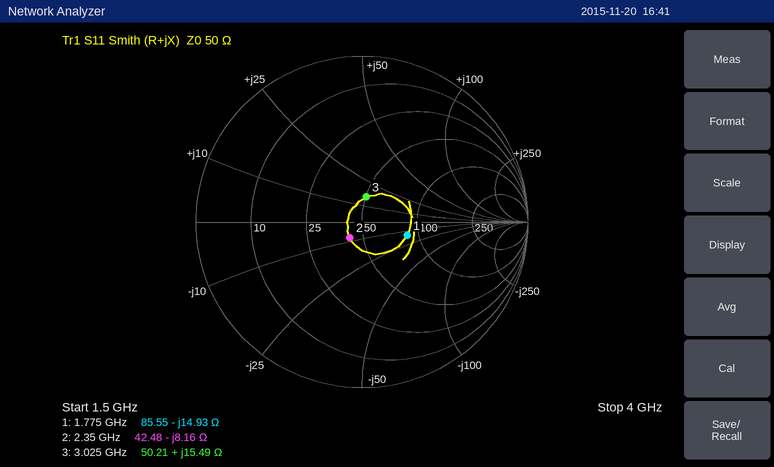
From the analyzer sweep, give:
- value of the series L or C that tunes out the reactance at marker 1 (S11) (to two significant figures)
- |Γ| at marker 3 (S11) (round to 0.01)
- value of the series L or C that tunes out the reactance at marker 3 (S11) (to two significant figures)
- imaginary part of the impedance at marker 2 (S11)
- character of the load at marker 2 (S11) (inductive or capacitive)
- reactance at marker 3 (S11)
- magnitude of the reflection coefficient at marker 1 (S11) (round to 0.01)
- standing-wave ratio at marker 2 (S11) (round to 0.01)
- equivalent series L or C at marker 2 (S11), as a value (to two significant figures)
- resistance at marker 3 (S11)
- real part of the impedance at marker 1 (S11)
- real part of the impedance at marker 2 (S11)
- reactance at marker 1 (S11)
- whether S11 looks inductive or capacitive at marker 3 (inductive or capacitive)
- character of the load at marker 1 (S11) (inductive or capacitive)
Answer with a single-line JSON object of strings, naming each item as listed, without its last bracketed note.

{"value of the series L or C that tunes out the reactance at marker 1 (S11)": "1.3 nH", "|Γ| at marker 3 (S11)": "0.15", "value of the series L or C that tunes out the reactance at marker 3 (S11)": "3.4 pF", "imaginary part of the impedance at marker 2": "-8.16 Ω", "character of the load at marker 2 (S11)": "capacitive", "reactance at marker 3": "+15.49 Ω", "magnitude of the reflection coefficient at marker 1 (S11)": "0.28", "standing-wave ratio at marker 2 (S11)": "1.27", "equivalent series L or C at marker 2 (S11), as a value": "8.3 pF", "resistance at marker 3": "50.21 Ω", "real part of the impedance at marker 1": "85.55 Ω", "real part of the impedance at marker 2": "42.48 Ω", "reactance at marker 1": "-14.93 Ω", "whether S11 looks inductive or capacitive at marker 3": "inductive", "character of the load at marker 1 (S11)": "capacitive"}
